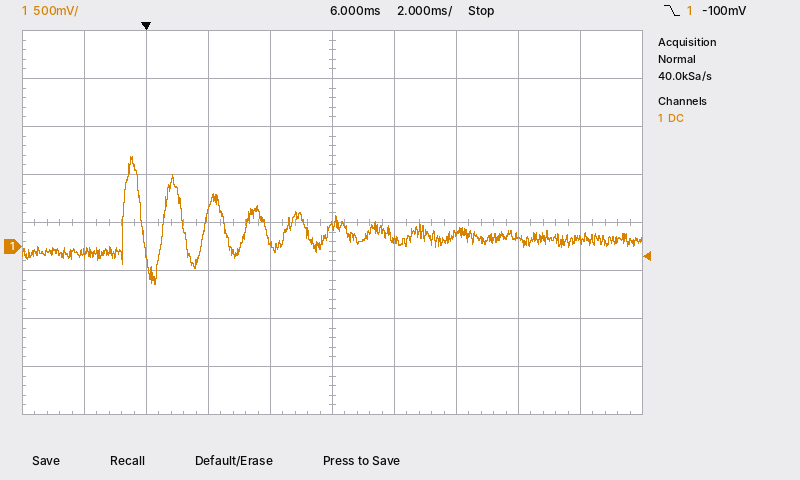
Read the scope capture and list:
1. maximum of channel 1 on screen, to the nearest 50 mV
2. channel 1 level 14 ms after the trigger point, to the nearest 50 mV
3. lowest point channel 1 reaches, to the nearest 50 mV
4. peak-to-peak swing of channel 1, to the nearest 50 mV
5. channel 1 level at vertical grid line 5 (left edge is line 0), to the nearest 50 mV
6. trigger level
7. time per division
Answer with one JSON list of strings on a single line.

["950 mV", "50 mV", "-400 mV", "1.35 V", "200 mV", "-100 mV", "2 ms"]
